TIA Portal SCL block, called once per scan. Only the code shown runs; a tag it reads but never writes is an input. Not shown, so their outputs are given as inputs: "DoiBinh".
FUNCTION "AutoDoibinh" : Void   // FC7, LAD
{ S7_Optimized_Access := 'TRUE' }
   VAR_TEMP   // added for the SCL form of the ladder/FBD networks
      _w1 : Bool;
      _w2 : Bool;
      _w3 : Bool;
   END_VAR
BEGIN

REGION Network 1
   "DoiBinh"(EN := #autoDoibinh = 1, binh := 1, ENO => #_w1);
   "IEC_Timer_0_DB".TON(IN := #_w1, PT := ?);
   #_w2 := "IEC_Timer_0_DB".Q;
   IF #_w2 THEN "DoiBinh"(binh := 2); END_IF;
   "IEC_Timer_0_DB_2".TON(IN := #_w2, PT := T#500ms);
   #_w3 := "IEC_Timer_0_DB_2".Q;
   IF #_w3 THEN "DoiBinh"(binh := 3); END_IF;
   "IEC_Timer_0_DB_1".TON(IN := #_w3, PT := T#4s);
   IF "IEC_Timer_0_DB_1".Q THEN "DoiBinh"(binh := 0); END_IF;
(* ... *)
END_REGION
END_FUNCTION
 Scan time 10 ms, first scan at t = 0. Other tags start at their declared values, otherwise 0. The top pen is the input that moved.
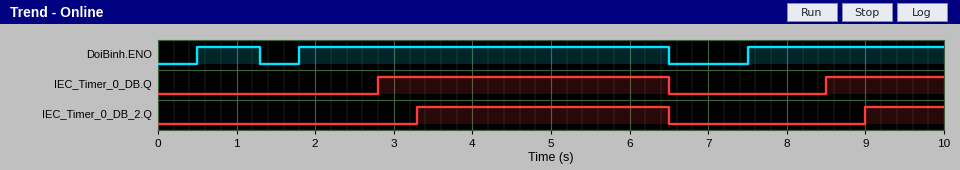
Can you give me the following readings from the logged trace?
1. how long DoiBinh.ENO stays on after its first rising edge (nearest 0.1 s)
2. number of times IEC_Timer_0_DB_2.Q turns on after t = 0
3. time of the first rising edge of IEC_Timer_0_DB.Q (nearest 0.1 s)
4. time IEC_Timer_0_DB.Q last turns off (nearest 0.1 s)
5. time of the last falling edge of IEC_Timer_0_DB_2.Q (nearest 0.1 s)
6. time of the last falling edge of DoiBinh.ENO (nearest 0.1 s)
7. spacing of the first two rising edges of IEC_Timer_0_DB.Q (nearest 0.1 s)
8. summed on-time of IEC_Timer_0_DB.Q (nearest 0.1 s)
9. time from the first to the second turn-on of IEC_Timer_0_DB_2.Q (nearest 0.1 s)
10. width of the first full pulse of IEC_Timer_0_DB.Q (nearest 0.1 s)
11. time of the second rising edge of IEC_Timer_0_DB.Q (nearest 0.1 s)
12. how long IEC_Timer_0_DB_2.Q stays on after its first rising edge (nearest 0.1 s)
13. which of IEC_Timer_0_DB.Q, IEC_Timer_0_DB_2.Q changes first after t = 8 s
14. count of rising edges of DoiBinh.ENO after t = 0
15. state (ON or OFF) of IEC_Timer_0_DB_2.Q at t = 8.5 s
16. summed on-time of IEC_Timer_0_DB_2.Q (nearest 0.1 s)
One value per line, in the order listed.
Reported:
0.8 s
2
2.8 s
6.5 s
6.5 s
6.5 s
5.7 s
5.2 s
5.7 s
3.7 s
8.5 s
3.2 s
IEC_Timer_0_DB.Q
3
OFF
4.2 s
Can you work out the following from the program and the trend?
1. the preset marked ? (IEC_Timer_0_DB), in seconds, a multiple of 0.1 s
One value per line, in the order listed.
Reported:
1.0 s
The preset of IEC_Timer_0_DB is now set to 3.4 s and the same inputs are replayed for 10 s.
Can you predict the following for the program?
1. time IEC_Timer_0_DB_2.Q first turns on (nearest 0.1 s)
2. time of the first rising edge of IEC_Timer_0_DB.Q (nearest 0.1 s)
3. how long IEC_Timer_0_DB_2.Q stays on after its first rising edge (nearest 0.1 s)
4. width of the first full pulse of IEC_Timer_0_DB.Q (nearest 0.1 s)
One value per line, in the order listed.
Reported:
5.7 s
5.2 s
0.8 s
1.3 s
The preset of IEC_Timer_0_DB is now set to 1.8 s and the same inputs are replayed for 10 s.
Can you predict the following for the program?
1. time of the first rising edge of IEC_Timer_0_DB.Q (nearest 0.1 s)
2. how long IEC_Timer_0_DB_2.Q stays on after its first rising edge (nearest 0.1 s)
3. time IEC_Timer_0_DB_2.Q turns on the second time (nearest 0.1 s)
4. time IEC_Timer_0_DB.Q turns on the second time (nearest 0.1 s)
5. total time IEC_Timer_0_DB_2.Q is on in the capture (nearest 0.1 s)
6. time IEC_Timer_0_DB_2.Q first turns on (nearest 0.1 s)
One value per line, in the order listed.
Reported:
3.6 s
2.4 s
9.8 s
9.3 s
2.6 s
4.1 s
